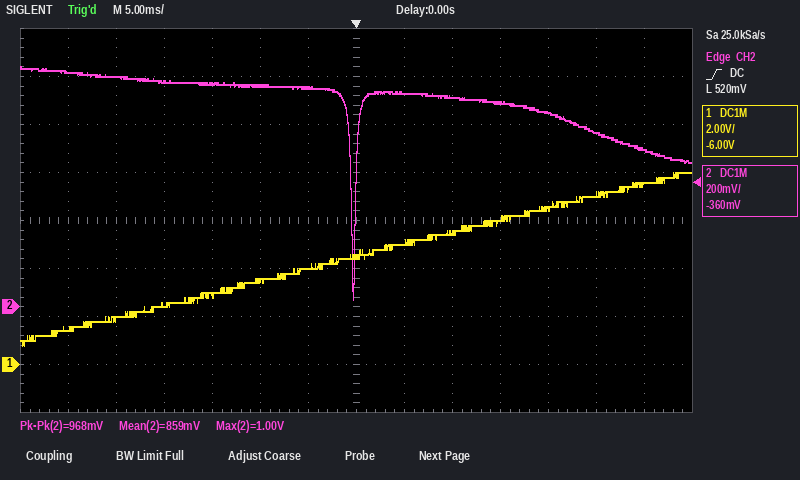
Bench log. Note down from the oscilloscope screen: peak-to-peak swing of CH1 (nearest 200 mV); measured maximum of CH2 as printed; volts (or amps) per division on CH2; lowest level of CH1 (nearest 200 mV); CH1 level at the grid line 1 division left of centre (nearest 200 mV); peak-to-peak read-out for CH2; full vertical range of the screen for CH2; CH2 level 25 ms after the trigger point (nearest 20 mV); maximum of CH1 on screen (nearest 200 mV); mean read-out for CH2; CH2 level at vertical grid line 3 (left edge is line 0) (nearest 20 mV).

7.2 V
1.00 V
200 mV
800 mV
4.0 V
968 mV
1.6 V
720 mV
8.0 V
859 mV
940 mV
